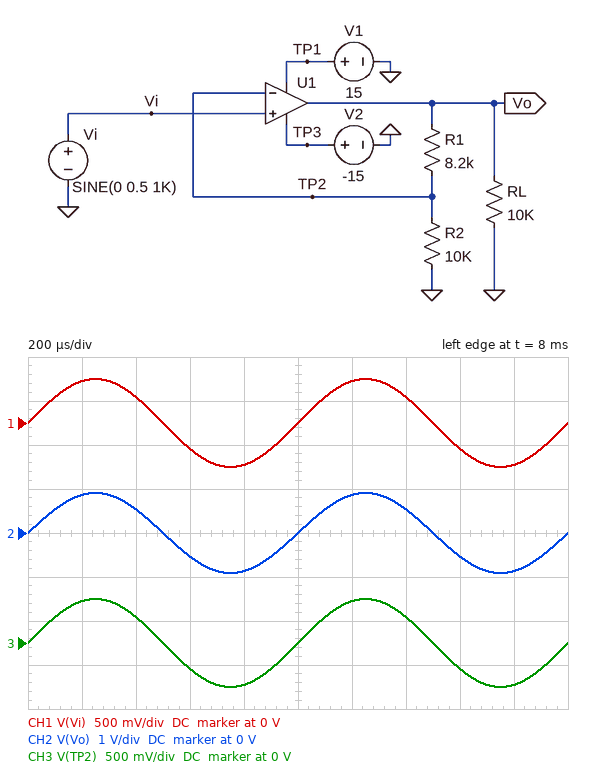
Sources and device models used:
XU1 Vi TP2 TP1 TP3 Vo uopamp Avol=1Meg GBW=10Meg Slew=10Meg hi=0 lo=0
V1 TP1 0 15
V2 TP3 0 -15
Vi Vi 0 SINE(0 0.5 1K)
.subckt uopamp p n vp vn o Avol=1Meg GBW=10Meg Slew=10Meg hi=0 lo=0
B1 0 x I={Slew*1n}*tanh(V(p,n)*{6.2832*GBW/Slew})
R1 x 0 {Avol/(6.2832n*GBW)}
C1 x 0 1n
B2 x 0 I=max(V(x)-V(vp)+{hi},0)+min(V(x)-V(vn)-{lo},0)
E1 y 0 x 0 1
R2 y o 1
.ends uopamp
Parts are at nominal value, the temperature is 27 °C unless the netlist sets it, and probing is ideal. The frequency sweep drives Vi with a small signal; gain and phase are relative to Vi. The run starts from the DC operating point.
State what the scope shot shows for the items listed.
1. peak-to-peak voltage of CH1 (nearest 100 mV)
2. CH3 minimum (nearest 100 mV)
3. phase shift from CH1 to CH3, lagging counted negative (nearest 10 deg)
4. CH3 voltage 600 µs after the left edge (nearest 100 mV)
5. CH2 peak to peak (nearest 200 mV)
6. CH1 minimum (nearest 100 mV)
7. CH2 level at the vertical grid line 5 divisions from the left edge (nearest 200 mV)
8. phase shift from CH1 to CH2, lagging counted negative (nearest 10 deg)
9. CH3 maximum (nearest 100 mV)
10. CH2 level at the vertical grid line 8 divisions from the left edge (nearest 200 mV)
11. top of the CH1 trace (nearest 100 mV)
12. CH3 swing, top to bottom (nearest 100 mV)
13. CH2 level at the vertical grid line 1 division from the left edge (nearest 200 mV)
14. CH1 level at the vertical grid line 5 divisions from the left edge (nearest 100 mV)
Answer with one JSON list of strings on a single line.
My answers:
["1.0 V", "-500 mV", "0 deg", "-300 mV", "1.8 V", "-500 mV", "0 V", "0 deg", "500 mV", "-600 mV", "500 mV", "1.0 V", "800 mV", "0 V"]
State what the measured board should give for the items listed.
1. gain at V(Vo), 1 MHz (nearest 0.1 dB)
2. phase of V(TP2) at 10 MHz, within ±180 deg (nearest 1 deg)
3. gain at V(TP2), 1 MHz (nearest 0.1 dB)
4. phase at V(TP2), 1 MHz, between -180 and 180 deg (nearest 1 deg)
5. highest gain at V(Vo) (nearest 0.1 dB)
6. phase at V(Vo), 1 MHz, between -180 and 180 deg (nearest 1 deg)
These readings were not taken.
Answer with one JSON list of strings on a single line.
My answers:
["5.1 dB", "-61 deg", "-0.1 dB", "-10 deg", "5.2 dB", "-10 deg"]
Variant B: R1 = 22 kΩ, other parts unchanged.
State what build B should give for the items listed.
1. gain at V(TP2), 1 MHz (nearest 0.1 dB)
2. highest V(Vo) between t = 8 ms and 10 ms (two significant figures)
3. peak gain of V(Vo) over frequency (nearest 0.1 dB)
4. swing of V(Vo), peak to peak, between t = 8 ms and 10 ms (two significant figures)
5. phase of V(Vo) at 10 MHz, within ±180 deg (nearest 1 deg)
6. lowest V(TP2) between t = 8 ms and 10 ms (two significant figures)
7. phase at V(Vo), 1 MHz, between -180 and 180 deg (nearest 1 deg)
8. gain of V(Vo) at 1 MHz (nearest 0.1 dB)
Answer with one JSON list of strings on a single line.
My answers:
["-0.4 dB", "1.6 V", "10.1 dB", "3.2 V", "-73 deg", "-500 mV", "-18 deg", "9.7 dB"]
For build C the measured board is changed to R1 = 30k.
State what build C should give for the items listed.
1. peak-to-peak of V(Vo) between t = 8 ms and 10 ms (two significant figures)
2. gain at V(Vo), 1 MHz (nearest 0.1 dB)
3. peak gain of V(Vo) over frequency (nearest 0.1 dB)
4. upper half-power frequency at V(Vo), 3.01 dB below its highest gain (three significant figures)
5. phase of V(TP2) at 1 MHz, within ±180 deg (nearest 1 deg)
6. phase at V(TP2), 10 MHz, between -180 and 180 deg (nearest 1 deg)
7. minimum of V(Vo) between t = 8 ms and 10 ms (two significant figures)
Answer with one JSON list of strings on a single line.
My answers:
["4.0 V", "11.4 dB", "12.0 dB", "2.50 MHz", "-22 deg", "-76 deg", "-2.0 V"]
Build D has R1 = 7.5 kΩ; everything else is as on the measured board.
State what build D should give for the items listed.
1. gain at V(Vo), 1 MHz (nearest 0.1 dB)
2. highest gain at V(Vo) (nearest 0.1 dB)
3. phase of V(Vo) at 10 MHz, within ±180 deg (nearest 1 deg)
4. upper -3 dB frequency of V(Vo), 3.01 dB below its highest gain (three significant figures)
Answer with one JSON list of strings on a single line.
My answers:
["4.7 dB", "4.9 dB", "-60 deg", "5.71 MHz"]
